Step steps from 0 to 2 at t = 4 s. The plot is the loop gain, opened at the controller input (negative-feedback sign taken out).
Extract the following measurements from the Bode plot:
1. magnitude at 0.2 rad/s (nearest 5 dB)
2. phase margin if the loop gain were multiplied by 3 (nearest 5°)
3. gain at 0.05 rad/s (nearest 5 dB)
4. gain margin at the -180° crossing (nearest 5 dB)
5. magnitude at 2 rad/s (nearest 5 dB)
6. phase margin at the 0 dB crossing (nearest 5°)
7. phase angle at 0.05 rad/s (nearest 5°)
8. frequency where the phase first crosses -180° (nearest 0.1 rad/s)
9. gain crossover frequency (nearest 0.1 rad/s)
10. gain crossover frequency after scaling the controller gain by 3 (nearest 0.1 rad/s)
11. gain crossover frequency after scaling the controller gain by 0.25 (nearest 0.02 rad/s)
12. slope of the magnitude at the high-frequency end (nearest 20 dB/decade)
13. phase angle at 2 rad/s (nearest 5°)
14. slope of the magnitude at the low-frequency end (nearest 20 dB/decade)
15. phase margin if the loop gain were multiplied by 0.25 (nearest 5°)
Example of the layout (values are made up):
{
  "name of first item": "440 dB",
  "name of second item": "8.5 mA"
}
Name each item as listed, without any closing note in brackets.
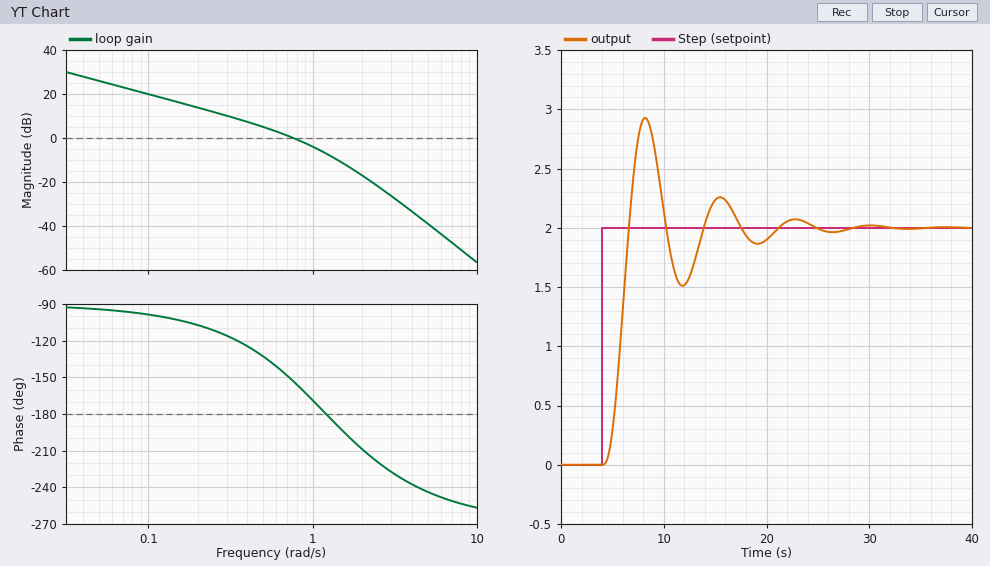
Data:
{
  "magnitude at 0.2 rad/s": "15 dB",
  "phase margin if the loop gain were multiplied by 3": "-10°",
  "gain at 0.05 rad/s": "25 dB",
  "gain margin at the -180° crossing": "5 dB",
  "magnitude at 2 rad/s": "-15 dB",
  "phase margin at the 0 dB crossing": "25°",
  "phase angle at 0.05 rad/s": "-95°",
  "frequency where the phase first crosses -180°": "1.2 rad/s",
  "gain crossover frequency": "0.8 rad/s",
  "gain crossover frequency after scaling the controller gain by 3": "1.4 rad/s",
  "gain crossover frequency after scaling the controller gain by 0.25": "0.24 rad/s",
  "slope of the magnitude at the high-frequency end": "-60 dB/decade",
  "phase angle at 2 rad/s": "-210°",
  "slope of the magnitude at the low-frequency end": "-20 dB/decade",
  "phase margin if the loop gain were multiplied by 0.25": "70°"
}
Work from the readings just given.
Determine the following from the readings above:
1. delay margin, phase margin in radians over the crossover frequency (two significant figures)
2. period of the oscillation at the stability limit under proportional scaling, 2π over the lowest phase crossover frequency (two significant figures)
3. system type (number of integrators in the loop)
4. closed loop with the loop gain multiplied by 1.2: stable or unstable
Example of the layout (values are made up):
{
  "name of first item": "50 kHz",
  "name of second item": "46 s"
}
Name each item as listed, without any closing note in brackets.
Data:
{
  "delay margin, phase margin in radians over the crossover frequency": "0.55 s",
  "period of the oscillation at the stability limit under proportional scaling, 2π over the lowest phase crossover frequency": "5.2 s",
  "system type": "1",
  "closed loop with the loop gain multiplied by 1.2: stable or unstable": "stable"
}
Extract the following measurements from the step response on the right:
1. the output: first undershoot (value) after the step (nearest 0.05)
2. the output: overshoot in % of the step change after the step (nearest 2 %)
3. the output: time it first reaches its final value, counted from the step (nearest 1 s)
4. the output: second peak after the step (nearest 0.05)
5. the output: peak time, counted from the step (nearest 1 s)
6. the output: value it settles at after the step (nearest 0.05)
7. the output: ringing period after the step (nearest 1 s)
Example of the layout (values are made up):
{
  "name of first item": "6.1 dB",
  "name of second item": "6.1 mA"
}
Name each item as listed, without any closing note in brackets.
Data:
{
  "the output: first undershoot (value) after the step": "1.50",
  "the output: overshoot in % of the step change after the step": "46 %",
  "the output: time it first reaches its final value, counted from the step": "3 s",
  "the output: second peak after the step": "2.25",
  "the output: peak time, counted from the step": "4 s",
  "the output: value it settles at after the step": "2.00",
  "the output: ringing period after the step": "7 s"
}
